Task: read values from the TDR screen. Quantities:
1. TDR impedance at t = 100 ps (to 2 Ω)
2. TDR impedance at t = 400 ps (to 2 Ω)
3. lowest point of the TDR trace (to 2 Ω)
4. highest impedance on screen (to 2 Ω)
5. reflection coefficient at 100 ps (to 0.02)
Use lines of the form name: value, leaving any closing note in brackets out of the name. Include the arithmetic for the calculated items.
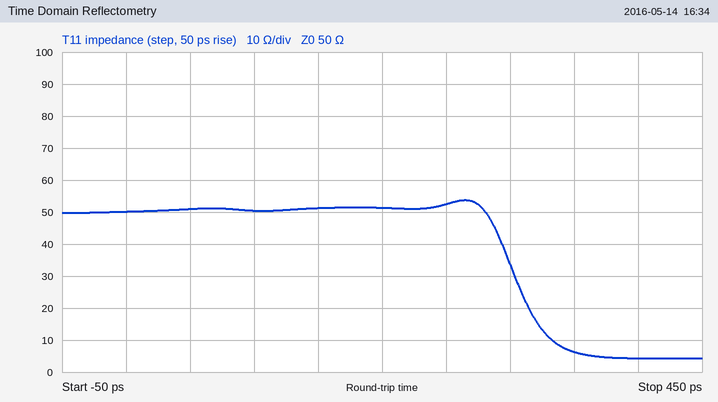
TDR impedance at t = 100 ps: 50 Ω
TDR impedance at t = 400 ps: 4 Ω
lowest point of the TDR trace: 4 Ω
highest impedance on screen: 54 Ω
reflection coefficient at 100 ps: (50 − 50)/(50 + 50) ≈ 0.00
